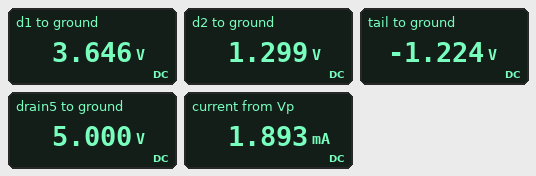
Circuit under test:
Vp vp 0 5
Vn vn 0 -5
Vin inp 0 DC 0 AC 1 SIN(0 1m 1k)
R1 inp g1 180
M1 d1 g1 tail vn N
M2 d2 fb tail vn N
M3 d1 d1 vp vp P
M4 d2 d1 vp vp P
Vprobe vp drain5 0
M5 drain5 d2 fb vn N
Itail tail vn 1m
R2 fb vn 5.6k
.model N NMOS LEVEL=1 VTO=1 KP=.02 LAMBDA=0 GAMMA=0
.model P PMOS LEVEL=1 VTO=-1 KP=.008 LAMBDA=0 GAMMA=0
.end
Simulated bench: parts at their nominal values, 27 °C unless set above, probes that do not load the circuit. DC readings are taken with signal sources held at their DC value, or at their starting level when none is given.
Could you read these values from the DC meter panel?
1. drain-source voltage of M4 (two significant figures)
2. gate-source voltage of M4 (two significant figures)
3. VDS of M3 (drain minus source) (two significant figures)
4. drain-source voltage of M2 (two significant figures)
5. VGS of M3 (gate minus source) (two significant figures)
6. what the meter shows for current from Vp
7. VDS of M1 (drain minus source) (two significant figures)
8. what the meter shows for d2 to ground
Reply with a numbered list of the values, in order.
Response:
1. -3.7 V
2. -1.4 V
3. -1.4 V
4. 2.5 V
5. -1.4 V
6. 1.893 mA
7. 4.9 V
8. 1.299 V
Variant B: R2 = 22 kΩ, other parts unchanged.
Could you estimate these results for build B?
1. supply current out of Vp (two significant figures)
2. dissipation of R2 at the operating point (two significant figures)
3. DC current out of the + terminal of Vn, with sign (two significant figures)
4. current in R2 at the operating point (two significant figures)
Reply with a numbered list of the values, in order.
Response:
1. 1.2 mA
2. 1.1 mW
3. -1.2 mA
4. 230 µA
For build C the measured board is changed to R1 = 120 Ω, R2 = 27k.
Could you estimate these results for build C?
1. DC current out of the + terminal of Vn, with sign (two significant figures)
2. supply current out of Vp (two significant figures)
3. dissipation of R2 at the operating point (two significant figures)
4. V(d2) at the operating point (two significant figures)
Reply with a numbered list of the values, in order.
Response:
1. -1.2 mA
2. 1.2 mA
3. 930 µW
4. 1.1 V
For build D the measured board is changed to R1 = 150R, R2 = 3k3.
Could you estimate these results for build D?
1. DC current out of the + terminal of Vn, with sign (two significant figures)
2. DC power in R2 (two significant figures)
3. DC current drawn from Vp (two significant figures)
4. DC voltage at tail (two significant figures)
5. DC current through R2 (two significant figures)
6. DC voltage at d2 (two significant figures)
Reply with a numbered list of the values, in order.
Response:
1. -2.5 mA
2. 7.6 mW
3. 2.5 mA
4. -1.2 V
5. 1.5 mA
6. 1.4 V
